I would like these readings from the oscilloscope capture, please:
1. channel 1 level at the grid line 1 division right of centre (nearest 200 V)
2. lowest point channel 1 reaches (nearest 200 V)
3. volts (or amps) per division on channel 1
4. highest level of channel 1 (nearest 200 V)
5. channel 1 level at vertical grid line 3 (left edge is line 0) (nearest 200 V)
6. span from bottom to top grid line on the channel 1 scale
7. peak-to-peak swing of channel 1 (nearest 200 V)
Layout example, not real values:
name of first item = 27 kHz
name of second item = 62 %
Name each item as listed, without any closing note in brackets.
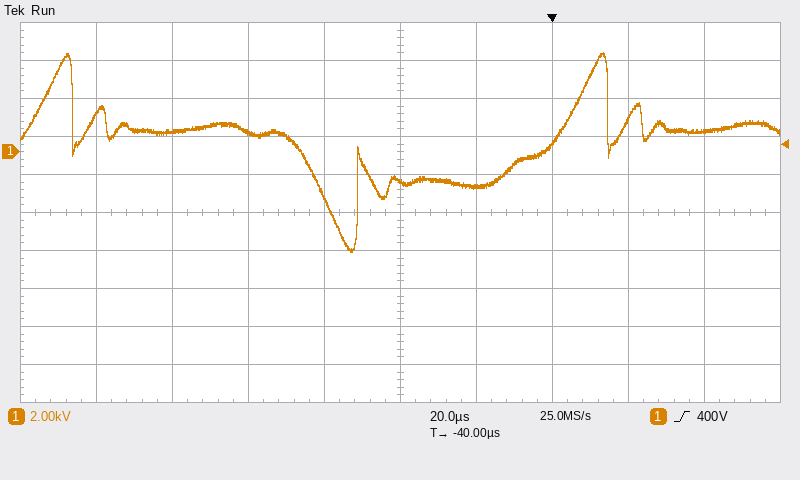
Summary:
channel 1 level at the grid line 1 division right of centre = -1.8 kV
lowest point channel 1 reaches = -5.2 kV
volts (or amps) per division on channel 1 = 2 kV
highest level of channel 1 = 5.2 kV
channel 1 level at vertical grid line 3 (left edge is line 0) = 1.0 kV
span from bottom to top grid line on the channel 1 scale = 20 kV
peak-to-peak swing of channel 1 = 10.4 kV
